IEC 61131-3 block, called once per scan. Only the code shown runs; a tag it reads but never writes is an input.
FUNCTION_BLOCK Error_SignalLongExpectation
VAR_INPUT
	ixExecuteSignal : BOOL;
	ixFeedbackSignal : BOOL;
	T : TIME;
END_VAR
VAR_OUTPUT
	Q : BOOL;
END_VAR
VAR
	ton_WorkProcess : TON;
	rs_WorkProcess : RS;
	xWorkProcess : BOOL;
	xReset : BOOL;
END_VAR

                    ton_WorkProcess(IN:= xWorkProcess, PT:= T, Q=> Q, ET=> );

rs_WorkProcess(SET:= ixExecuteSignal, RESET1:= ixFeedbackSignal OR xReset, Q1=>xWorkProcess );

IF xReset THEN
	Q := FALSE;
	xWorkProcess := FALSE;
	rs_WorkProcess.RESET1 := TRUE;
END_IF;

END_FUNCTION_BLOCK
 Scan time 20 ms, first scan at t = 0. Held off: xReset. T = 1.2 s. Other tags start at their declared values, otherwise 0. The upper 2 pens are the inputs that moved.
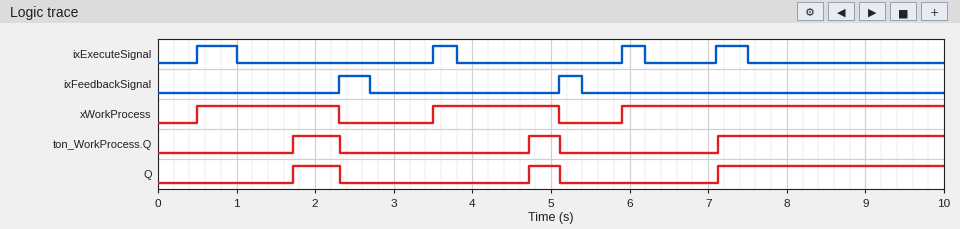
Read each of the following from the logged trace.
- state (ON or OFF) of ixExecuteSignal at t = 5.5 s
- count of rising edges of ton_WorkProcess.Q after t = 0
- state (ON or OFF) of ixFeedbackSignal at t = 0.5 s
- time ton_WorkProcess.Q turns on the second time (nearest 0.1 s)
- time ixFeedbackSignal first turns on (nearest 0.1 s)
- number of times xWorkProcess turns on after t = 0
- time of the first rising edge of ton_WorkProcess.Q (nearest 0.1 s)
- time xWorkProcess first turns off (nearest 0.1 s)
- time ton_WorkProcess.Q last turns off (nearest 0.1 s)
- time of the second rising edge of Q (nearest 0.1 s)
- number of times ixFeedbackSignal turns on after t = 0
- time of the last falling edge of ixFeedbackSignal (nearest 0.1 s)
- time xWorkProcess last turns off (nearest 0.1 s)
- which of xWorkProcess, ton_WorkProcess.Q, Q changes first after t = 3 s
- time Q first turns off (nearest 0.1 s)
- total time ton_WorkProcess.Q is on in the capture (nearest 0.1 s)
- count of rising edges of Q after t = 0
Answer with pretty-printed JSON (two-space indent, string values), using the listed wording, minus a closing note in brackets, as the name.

{
  "state (ON or OFF) of ixExecuteSignal at t = 5.5 s": "OFF",
  "count of rising edges of ton_WorkProcess.Q after t = 0": "3",
  "state (ON or OFF) of ixFeedbackSignal at t = 0.5 s": "OFF",
  "time ton_WorkProcess.Q turns on the second time": "4.7 s",
  "time ixFeedbackSignal first turns on": "2.3 s",
  "number of times xWorkProcess turns on after t = 0": "3",
  "time of the first rising edge of ton_WorkProcess.Q": "1.7 s",
  "time xWorkProcess first turns off": "2.3 s",
  "time ton_WorkProcess.Q last turns off": "5.1 s",
  "time of the second rising edge of Q": "4.7 s",
  "number of times ixFeedbackSignal turns on after t = 0": "2",
  "time of the last falling edge of ixFeedbackSignal": "5.4 s",
  "time xWorkProcess last turns off": "5.1 s",
  "which of xWorkProcess, ton_WorkProcess.Q, Q changes first after t = 3 s": "xWorkProcess",
  "time Q first turns off": "2.3 s",
  "total time ton_WorkProcess.Q is on in the capture": "3.9 s",
  "count of rising edges of Q after t = 0": "3"
}
